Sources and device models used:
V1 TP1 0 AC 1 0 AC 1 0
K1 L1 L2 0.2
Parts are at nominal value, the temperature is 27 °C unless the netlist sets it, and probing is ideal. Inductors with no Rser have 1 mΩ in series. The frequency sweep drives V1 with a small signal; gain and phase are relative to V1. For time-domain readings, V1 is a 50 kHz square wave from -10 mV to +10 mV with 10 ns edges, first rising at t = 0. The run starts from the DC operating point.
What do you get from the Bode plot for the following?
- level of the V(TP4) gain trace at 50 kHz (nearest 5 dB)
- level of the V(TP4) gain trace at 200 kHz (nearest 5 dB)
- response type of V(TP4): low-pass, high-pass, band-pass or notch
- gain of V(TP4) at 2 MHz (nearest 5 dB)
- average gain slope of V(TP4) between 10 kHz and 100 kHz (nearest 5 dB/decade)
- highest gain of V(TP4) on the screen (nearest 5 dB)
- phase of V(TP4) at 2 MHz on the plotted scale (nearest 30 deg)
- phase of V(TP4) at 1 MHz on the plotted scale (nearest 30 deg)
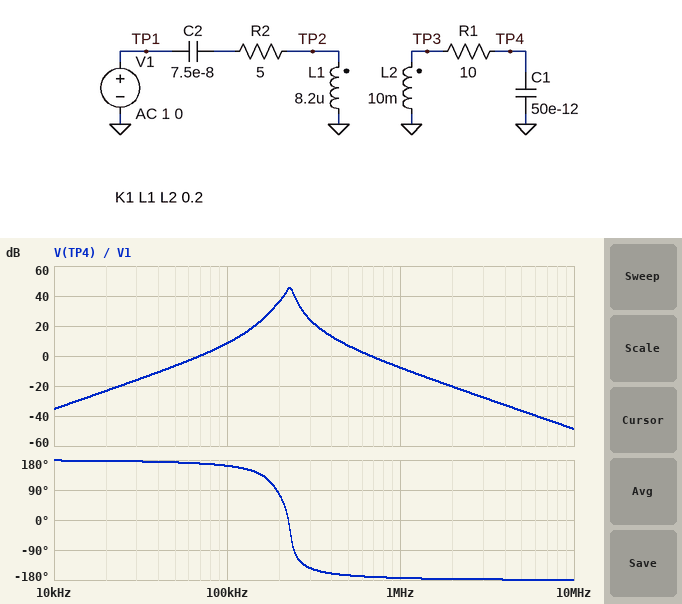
-5 dB
35 dB
band-pass
-20 dB
45 dB/decade
45 dB
-180 deg
-180 deg
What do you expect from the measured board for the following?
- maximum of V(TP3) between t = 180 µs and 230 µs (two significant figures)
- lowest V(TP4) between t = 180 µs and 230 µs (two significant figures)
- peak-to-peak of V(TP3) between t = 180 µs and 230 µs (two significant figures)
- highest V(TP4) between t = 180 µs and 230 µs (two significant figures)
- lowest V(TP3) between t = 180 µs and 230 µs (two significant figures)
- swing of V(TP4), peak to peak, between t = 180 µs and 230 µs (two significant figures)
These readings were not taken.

220 mV
-220 mV
440 mV
220 mV
-220 mV
440 mV
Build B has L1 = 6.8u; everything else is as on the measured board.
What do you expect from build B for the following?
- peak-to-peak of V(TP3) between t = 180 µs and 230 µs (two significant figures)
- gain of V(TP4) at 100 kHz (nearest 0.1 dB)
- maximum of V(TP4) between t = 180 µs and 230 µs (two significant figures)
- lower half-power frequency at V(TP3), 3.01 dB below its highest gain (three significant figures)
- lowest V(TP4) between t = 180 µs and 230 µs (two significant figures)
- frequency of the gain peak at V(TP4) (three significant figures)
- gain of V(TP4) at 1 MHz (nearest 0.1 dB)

400 mV
7.3 dB
200 mV
215 kHz
-200 mV
225 kHz
-7.0 dB
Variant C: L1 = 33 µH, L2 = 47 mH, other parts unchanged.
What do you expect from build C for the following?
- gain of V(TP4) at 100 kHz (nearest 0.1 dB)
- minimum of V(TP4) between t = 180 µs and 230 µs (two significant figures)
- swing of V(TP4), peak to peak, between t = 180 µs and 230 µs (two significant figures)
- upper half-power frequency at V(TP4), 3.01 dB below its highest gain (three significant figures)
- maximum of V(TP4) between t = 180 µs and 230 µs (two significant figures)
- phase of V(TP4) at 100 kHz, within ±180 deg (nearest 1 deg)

45.6 dB
-87 mV
170 mV
116 kHz
87 mV
26 deg
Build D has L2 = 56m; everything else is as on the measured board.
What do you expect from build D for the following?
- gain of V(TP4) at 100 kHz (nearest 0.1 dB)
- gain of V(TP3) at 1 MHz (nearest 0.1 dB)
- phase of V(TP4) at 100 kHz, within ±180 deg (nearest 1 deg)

32.6 dB
-15.7 dB
-15 deg
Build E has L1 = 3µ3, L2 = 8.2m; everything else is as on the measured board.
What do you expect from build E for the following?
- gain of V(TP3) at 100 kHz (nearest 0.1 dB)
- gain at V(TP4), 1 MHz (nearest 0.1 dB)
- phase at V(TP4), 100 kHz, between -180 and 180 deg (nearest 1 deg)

1.9 dB
-2.6 dB
165 deg
